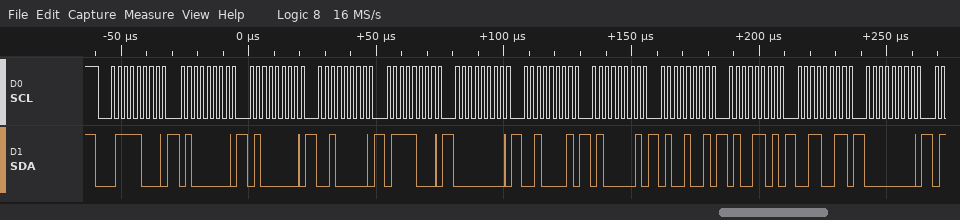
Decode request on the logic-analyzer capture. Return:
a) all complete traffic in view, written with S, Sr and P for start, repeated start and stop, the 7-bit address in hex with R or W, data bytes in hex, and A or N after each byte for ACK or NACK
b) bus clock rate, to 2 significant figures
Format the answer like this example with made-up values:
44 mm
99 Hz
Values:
S 3CW A 40 A 40 A 20 A 78 A 00 A 21 A 41 A 49 A 4D A 33 A 00 A
400 kHz
